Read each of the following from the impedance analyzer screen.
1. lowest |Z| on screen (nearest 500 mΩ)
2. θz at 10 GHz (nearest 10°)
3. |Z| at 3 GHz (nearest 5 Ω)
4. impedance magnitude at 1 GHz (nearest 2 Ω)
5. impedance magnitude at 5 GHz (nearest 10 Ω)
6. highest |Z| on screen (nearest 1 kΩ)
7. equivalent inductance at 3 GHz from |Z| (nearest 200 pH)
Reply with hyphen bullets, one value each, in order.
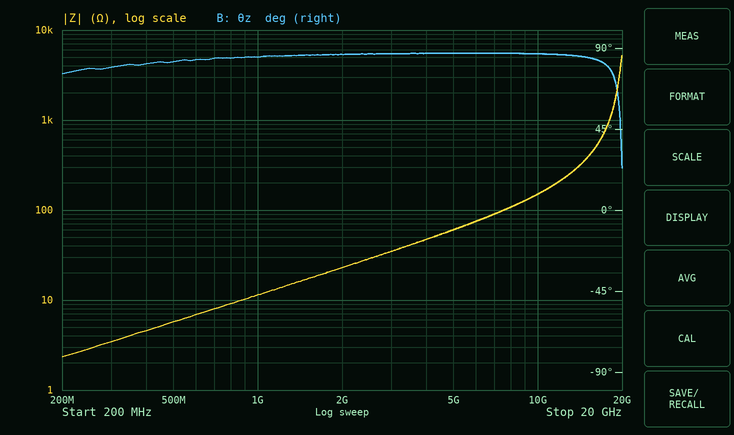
- 2.5 Ω
- 90°
- 35 Ω
- 12 Ω
- 60 Ω
- 5 kΩ
- 1.8 nH
